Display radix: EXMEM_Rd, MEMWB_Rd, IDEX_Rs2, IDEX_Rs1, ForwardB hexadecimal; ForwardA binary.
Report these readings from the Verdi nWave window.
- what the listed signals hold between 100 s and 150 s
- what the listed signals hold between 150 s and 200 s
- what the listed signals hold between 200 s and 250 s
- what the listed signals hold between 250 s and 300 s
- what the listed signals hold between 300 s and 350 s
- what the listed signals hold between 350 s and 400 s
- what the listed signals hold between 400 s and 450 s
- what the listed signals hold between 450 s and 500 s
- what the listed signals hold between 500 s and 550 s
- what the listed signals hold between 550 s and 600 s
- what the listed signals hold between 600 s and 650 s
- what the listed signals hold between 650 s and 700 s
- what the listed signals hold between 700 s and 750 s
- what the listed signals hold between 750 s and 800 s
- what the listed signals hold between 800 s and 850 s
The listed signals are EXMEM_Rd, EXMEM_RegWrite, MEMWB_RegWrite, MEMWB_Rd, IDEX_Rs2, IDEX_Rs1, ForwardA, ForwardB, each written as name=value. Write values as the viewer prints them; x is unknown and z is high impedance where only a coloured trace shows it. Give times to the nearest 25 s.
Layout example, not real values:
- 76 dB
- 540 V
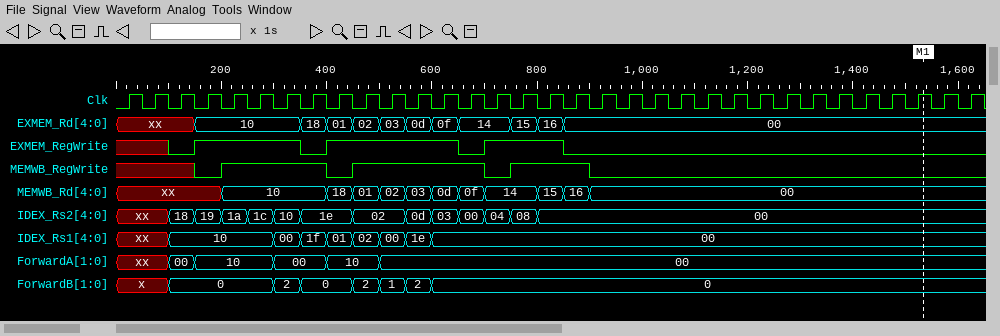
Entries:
- EXMEM_Rd=xx, EXMEM_RegWrite=0, MEMWB_RegWrite=x, MEMWB_Rd=xx, IDEX_Rs2=18, IDEX_Rs1=10, ForwardA=00, ForwardB=0
- EXMEM_Rd=10, EXMEM_RegWrite=1, MEMWB_RegWrite=0, MEMWB_Rd=xx, IDEX_Rs2=19, IDEX_Rs1=10, ForwardA=10, ForwardB=0
- EXMEM_Rd=10, EXMEM_RegWrite=1, MEMWB_RegWrite=1, MEMWB_Rd=10, IDEX_Rs2=1a, IDEX_Rs1=10, ForwardA=10, ForwardB=0
- EXMEM_Rd=10, EXMEM_RegWrite=1, MEMWB_RegWrite=1, MEMWB_Rd=10, IDEX_Rs2=1c, IDEX_Rs1=10, ForwardA=10, ForwardB=0
- EXMEM_Rd=10, EXMEM_RegWrite=1, MEMWB_RegWrite=1, MEMWB_Rd=10, IDEX_Rs2=10, IDEX_Rs1=00, ForwardA=00, ForwardB=2
- EXMEM_Rd=18, EXMEM_RegWrite=0, MEMWB_RegWrite=1, MEMWB_Rd=10, IDEX_Rs2=1e, IDEX_Rs1=1f, ForwardA=00, ForwardB=0
- EXMEM_Rd=01, EXMEM_RegWrite=1, MEMWB_RegWrite=0, MEMWB_Rd=18, IDEX_Rs2=1e, IDEX_Rs1=01, ForwardA=10, ForwardB=0
- EXMEM_Rd=02, EXMEM_RegWrite=1, MEMWB_RegWrite=1, MEMWB_Rd=01, IDEX_Rs2=02, IDEX_Rs1=02, ForwardA=10, ForwardB=2
- EXMEM_Rd=03, EXMEM_RegWrite=1, MEMWB_RegWrite=1, MEMWB_Rd=02, IDEX_Rs2=02, IDEX_Rs1=00, ForwardA=00, ForwardB=1
- EXMEM_Rd=0d, EXMEM_RegWrite=1, MEMWB_RegWrite=1, MEMWB_Rd=03, IDEX_Rs2=0d, IDEX_Rs1=1e, ForwardA=00, ForwardB=2
- EXMEM_Rd=0f, EXMEM_RegWrite=1, MEMWB_RegWrite=1, MEMWB_Rd=0d, IDEX_Rs2=03, IDEX_Rs1=00, ForwardA=00, ForwardB=0
- EXMEM_Rd=14, EXMEM_RegWrite=0, MEMWB_RegWrite=1, MEMWB_Rd=0f, IDEX_Rs2=00, IDEX_Rs1=00, ForwardA=00, ForwardB=0
- EXMEM_Rd=14, EXMEM_RegWrite=1, MEMWB_RegWrite=0, MEMWB_Rd=14, IDEX_Rs2=04, IDEX_Rs1=00, ForwardA=00, ForwardB=0
- EXMEM_Rd=15, EXMEM_RegWrite=1, MEMWB_RegWrite=1, MEMWB_Rd=14, IDEX_Rs2=08, IDEX_Rs1=00, ForwardA=00, ForwardB=0
- EXMEM_Rd=16, EXMEM_RegWrite=1, MEMWB_RegWrite=1, MEMWB_Rd=15, IDEX_Rs2=00, IDEX_Rs1=00, ForwardA=00, ForwardB=0
